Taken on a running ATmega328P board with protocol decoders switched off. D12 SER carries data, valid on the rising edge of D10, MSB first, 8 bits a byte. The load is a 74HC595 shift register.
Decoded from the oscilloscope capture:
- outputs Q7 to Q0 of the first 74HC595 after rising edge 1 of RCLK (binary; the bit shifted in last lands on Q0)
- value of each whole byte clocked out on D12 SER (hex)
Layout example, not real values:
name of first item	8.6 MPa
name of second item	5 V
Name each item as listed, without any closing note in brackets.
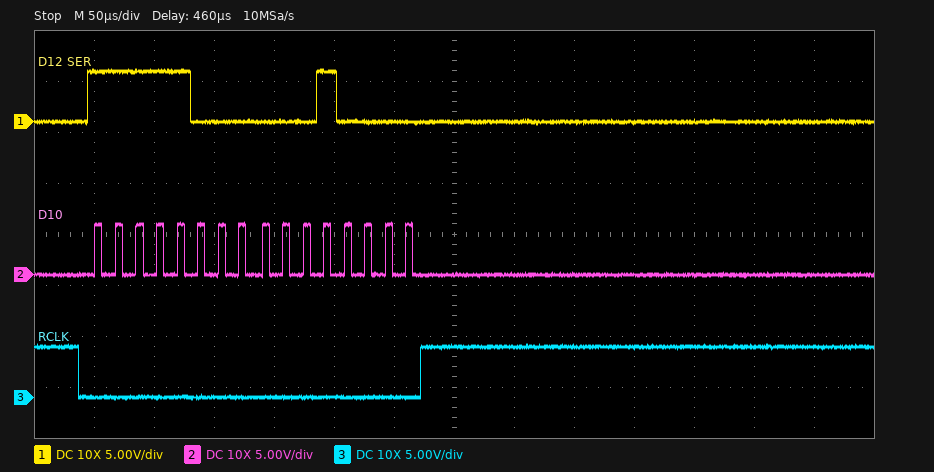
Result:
outputs Q7 to Q0 of the first 74HC595 after rising edge 1 of RCLK	00010000
value of each whole byte clocked out on D12 SER	F8 10
